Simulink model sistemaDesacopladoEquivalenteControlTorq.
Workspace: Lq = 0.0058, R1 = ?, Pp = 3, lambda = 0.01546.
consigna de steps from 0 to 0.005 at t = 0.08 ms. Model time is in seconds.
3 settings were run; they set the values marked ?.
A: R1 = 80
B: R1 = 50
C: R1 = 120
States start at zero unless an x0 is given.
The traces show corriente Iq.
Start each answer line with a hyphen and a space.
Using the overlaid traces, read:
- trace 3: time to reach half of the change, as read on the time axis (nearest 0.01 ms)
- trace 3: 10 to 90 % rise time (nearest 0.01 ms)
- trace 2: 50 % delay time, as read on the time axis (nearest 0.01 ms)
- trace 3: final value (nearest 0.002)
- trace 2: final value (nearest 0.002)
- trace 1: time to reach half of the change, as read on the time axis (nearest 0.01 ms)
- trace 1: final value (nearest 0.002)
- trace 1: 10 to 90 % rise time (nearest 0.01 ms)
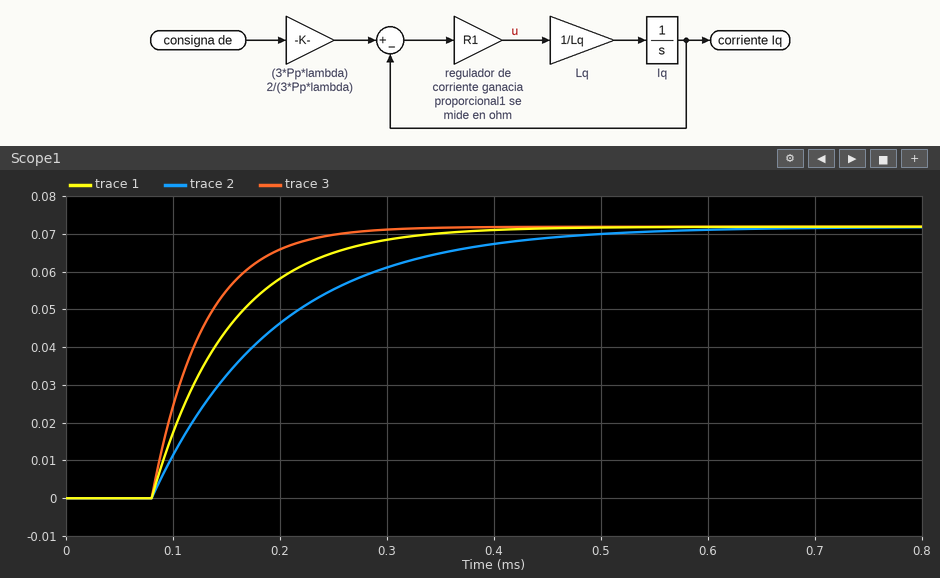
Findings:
- 0.11 ms
- 0.11 ms
- 0.16 ms
- 0.072
- 0.072
- 0.13 ms
- 0.072
- 0.16 ms
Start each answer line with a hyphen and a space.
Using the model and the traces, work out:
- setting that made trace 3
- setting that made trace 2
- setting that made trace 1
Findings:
- C
- B
- A
